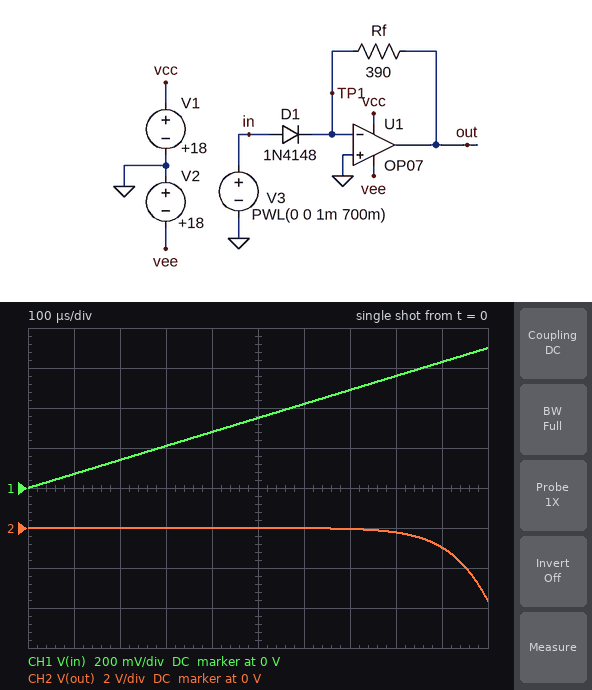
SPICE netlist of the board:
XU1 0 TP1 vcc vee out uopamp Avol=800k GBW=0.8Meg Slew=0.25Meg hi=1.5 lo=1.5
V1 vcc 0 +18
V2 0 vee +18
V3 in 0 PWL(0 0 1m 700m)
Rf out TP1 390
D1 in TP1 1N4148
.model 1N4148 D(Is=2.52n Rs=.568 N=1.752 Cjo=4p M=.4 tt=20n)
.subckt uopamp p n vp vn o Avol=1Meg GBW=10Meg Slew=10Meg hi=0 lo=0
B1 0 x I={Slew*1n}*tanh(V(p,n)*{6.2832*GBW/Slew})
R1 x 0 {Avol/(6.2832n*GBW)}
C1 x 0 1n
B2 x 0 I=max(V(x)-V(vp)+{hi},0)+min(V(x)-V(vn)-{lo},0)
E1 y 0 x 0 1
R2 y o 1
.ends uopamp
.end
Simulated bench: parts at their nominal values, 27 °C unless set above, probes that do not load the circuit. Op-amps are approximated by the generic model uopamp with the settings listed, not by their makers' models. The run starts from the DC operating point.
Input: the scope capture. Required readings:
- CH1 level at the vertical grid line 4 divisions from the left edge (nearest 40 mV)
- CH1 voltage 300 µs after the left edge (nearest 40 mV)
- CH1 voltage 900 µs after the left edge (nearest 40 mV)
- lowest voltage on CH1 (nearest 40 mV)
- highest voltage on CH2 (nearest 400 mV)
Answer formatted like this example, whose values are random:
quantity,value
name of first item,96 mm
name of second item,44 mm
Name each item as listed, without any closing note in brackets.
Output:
quantity,value
CH1 level at the vertical grid line 4 divisions from the left edge,280 mV
CH1 voltage 300 µs after the left edge,200 mV
CH1 voltage 900 µs after the left edge,640 mV
lowest voltage on CH1,0 V
highest voltage on CH2,0 V
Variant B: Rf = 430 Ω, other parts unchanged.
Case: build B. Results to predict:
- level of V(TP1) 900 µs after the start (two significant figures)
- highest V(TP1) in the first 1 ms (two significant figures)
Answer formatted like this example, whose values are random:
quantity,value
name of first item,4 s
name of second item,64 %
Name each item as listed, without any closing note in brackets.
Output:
quantity,value
level of V(TP1) 900 µs after the start,3.0 mV
highest V(TP1) in the first 1 ms,9.6 mV
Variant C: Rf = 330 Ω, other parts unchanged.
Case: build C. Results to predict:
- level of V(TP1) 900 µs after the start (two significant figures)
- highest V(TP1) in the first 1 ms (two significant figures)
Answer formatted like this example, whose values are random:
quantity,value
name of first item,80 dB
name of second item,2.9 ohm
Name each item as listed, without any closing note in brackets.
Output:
quantity,value
level of V(TP1) 900 µs after the start,2.4 mV
highest V(TP1) in the first 1 ms,7.8 mV
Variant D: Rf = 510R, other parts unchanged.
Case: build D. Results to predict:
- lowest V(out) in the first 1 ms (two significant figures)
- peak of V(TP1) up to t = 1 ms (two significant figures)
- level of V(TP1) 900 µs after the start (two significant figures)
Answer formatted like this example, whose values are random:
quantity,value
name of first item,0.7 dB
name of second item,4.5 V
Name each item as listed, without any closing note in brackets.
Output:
quantity,value
lowest V(out) in the first 1 ms,-4.6 V
peak of V(TP1) up to t = 1 ms,11 mV
level of V(TP1) 900 µs after the start,3.5 mV
